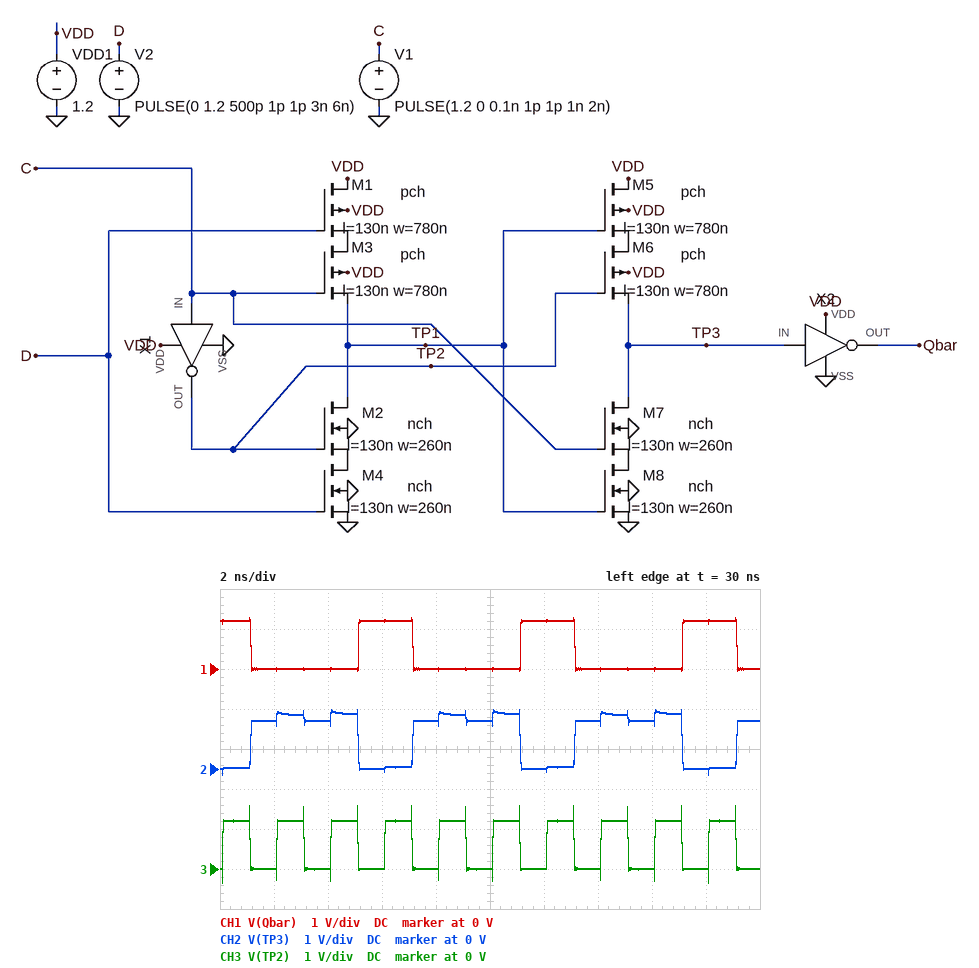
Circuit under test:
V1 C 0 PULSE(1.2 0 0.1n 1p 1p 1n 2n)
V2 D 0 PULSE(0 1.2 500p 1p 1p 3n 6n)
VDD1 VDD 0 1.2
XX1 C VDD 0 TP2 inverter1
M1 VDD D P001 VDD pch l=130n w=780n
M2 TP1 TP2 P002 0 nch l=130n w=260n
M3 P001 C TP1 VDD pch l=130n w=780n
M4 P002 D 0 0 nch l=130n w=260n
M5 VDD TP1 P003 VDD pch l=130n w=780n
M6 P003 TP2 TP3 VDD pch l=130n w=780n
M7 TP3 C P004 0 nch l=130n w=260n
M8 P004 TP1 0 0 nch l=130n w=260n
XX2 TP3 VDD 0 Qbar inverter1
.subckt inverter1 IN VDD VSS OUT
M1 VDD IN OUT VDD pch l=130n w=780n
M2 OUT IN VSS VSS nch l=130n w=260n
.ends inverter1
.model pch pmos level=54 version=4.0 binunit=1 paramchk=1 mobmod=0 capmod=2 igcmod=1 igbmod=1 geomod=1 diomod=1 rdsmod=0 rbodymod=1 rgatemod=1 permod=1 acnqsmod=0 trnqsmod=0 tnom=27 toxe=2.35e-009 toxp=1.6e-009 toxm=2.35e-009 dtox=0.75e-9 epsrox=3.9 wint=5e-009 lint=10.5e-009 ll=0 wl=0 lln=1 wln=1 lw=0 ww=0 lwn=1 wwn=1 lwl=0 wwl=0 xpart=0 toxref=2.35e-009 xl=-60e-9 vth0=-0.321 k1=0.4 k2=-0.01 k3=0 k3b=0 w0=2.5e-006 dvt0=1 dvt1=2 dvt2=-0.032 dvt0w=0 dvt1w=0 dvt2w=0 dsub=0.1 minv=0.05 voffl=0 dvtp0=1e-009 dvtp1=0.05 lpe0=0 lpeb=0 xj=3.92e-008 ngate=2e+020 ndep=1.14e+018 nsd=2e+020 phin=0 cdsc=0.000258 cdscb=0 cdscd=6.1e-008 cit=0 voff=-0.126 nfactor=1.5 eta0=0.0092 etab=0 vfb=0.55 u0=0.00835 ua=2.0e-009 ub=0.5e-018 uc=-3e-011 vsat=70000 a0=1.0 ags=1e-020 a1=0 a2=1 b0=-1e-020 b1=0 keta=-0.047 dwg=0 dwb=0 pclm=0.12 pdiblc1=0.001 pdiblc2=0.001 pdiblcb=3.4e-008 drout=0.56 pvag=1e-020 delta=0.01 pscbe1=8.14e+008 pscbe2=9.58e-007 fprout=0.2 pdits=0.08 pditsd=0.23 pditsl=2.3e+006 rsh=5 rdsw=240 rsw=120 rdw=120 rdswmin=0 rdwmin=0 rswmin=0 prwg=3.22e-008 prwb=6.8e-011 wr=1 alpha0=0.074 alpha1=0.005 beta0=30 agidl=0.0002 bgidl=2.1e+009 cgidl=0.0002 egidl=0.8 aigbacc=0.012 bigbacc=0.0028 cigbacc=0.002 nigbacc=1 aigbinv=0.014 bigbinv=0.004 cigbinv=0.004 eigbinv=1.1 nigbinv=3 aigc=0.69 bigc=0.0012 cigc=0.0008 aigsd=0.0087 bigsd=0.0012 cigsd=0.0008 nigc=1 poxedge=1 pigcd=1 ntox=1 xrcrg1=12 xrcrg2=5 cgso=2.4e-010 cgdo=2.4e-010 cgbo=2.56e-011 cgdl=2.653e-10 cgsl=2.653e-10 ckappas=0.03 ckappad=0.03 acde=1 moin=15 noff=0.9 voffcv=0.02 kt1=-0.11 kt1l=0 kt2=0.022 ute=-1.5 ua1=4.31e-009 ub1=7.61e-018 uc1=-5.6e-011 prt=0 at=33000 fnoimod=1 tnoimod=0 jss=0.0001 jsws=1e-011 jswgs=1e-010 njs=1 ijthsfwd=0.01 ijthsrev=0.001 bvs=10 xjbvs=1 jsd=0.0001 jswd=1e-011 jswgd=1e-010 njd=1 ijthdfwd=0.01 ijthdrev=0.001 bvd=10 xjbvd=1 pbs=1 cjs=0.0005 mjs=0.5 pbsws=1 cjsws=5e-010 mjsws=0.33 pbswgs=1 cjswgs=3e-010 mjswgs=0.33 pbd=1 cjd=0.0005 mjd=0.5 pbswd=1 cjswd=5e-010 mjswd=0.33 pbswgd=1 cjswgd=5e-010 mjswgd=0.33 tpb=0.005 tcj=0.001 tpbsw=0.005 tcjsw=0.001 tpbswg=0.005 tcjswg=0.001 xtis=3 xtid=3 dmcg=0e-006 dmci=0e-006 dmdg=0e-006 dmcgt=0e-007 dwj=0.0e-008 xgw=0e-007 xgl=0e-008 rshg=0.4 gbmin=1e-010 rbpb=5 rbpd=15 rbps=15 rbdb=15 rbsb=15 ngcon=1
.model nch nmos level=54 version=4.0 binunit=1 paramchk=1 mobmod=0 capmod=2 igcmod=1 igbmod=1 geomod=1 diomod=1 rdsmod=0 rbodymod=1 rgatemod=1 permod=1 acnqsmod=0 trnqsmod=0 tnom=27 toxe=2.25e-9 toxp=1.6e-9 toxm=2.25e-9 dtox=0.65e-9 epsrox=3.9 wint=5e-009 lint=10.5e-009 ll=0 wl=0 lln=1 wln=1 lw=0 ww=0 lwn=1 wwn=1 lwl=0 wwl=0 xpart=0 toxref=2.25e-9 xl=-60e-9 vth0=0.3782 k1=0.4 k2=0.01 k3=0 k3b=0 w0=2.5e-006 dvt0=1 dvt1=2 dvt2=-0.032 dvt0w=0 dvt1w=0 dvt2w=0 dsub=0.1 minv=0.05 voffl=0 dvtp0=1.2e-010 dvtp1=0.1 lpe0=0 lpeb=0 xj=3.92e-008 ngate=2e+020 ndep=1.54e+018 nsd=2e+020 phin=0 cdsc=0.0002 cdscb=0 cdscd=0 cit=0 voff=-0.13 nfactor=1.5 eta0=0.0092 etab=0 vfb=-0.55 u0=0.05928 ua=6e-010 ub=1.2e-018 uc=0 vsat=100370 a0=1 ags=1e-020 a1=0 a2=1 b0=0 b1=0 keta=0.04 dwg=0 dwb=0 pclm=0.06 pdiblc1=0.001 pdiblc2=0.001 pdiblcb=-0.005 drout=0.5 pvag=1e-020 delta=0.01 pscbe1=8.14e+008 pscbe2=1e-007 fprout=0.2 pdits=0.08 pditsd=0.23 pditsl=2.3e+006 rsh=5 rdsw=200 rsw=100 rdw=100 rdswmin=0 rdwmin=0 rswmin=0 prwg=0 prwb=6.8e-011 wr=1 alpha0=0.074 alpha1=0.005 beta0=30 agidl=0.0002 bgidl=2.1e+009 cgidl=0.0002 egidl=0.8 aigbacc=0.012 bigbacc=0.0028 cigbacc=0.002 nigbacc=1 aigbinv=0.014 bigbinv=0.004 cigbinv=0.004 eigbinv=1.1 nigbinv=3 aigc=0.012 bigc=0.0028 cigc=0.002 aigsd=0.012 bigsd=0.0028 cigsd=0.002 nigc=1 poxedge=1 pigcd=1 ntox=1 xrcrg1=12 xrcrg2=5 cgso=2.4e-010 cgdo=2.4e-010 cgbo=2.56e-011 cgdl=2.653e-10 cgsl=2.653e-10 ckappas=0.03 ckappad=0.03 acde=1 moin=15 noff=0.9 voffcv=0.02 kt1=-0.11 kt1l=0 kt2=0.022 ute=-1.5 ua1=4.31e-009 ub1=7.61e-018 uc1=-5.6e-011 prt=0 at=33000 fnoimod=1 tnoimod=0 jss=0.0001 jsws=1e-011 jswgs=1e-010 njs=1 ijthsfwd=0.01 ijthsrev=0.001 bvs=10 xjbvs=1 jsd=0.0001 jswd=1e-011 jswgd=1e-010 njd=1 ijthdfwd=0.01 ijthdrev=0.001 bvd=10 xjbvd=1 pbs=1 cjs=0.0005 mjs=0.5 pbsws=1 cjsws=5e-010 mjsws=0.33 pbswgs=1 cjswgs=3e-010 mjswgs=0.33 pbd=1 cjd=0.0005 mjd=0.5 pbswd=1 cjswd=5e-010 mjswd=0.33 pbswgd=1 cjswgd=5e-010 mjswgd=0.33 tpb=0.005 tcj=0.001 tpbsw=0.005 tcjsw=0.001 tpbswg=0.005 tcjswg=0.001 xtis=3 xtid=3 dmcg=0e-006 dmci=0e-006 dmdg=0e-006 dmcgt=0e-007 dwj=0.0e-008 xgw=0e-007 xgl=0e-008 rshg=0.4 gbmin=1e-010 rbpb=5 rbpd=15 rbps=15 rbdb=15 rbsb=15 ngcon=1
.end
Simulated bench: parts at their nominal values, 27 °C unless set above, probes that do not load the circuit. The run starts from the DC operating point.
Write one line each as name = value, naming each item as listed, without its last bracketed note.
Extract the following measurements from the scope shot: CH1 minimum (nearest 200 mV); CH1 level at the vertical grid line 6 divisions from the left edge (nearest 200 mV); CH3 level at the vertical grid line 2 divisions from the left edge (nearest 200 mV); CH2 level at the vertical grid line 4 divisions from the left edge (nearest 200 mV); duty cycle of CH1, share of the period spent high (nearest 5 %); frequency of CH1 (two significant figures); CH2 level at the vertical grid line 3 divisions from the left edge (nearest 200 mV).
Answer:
CH1 minimum = 0 V
CH1 level at the vertical grid line 6 divisions from the left edge = 1.2 V
CH3 level at the vertical grid line 2 divisions from the left edge = 0 V
CH2 level at the vertical grid line 4 divisions from the left edge = 1.2 V
duty cycle of CH1, share of the period spent high = 35 %
frequency of CH1 = 170 MHz
CH2 level at the vertical grid line 3 divisions from the left edge = 0 V
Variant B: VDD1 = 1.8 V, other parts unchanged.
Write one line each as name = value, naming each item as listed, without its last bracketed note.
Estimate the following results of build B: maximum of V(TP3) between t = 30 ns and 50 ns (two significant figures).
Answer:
maximum of V(TP3) between t = 30 ns and 50 ns = 1.7 V
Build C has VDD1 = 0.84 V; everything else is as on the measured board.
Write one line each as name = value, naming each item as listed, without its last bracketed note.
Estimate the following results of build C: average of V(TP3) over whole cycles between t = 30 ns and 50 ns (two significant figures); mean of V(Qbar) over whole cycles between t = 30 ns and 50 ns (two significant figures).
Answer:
average of V(TP3) over whole cycles between t = 30 ns and 50 ns = 610 mV
mean of V(Qbar) over whole cycles between t = 30 ns and 50 ns = 280 mV
